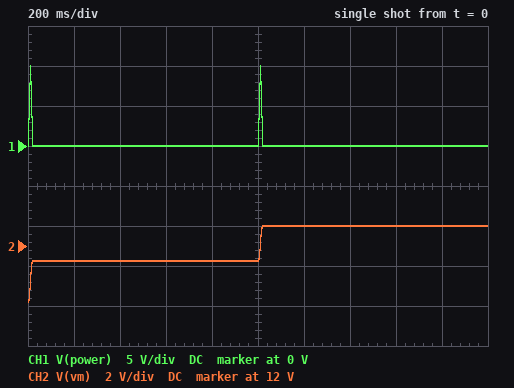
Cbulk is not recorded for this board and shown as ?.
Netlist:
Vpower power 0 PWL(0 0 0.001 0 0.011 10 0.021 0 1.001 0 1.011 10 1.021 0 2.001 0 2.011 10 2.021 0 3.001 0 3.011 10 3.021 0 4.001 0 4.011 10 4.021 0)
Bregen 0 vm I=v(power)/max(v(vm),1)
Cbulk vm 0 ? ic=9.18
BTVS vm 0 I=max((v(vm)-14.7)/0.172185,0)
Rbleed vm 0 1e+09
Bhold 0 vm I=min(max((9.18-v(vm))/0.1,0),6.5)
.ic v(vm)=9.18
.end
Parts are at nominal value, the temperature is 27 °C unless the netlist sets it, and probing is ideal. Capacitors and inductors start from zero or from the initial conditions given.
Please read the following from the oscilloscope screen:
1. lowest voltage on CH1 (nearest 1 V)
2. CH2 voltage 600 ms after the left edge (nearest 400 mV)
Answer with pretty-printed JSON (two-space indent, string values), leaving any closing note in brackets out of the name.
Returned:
{
  "lowest voltage on CH1": "0 V",
  "CH2 voltage 600 ms after the left edge": "11.2 V"
}
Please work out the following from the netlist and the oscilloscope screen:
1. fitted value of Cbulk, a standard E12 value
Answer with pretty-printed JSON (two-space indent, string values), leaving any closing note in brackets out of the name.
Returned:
{
  "fitted value of Cbulk, a standard E12 value": "4.7 mF"
}
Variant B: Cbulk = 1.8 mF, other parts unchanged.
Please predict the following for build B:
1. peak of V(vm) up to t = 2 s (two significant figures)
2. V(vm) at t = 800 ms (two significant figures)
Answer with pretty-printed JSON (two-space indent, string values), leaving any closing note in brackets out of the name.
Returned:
{
  "peak of V(vm) up to t = 2 s": "15 V",
  "V(vm) at t = 800 ms": "14 V"
}
